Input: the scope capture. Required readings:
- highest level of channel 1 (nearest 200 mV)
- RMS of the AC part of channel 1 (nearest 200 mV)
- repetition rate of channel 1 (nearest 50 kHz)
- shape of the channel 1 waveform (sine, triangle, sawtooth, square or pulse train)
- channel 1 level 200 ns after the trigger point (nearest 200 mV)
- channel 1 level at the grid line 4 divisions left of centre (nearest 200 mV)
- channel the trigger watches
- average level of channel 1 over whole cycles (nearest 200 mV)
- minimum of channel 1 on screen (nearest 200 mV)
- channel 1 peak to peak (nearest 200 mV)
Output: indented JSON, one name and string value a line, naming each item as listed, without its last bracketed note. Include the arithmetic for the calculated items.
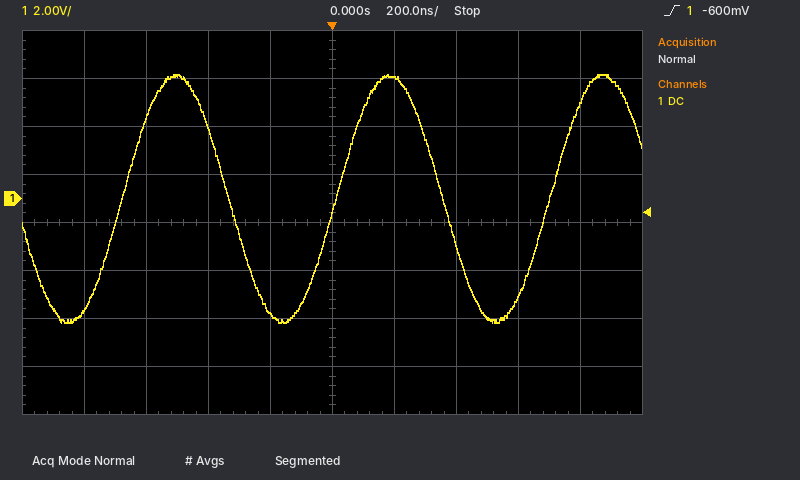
{
  "highest level of channel 1": "5.2 V",
  "RMS of the AC part of channel 1": "10.4 V / (2√2) ≈ 3.68 V, so 3.6 V to the nearest 200 mV",
  "repetition rate of channel 1": "1.45 MHz",
  "shape of the channel 1 waveform": "sine",
  "channel 1 level 200 ns after the trigger point": "5.0 V",
  "channel 1 level at the grid line 4 divisions left of centre": "-4.6 V",
  "channel the trigger watches": "channel 1",
  "average level of channel 1 over whole cycles": "(5.2 V + (-5.2 V)) / 2 ≈ 0.0 V",
  "minimum of channel 1 on screen": "-5.2 V",
  "channel 1 peak to peak": "5.2 V − (-5.2 V) = 10.4 V"
}
